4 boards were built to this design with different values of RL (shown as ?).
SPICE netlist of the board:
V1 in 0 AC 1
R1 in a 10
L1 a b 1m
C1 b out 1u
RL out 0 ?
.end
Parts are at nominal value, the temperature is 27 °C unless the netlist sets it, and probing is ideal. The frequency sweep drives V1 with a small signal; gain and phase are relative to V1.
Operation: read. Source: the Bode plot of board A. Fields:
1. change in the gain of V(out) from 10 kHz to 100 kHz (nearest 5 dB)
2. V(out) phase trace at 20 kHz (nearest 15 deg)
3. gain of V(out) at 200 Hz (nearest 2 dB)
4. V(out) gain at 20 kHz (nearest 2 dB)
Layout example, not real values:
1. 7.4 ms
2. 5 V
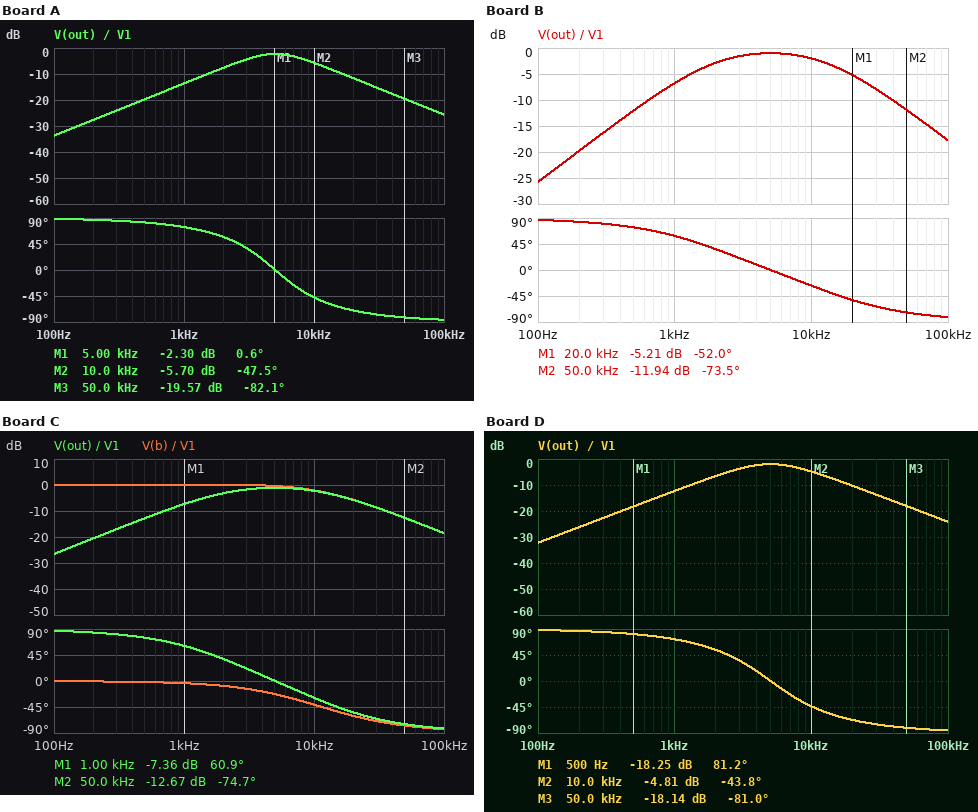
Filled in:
1. -20 dB
2. -75 deg
3. -28 dB
4. -12 dB
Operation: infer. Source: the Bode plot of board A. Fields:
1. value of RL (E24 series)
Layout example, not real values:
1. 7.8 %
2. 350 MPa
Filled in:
1. 33 Ω
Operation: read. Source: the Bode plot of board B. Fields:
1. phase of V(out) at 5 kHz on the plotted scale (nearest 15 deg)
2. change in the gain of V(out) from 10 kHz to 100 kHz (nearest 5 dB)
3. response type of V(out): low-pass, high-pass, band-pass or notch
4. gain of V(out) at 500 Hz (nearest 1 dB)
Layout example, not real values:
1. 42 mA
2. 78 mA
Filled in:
1. 0 deg
2. -15 dB
3. band-pass
4. -12 dB
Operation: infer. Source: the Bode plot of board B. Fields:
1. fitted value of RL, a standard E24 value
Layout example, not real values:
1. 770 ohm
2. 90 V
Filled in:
1. 82 Ω
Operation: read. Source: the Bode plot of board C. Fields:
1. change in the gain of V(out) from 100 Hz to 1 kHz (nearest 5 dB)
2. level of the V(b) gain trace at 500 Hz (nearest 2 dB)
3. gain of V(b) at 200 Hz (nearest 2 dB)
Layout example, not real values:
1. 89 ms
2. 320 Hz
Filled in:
1. 20 dB
2. 0 dB
3. 0 dB
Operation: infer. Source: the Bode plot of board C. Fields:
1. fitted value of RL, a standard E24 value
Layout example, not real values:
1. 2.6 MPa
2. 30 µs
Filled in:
1. 75 Ω
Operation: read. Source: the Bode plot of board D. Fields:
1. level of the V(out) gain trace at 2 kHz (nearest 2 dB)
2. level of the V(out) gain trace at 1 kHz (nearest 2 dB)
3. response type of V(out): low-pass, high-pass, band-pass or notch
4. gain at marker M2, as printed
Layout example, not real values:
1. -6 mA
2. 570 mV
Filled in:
1. -6 dB
2. -12 dB
3. band-pass
4. -4.81 dB
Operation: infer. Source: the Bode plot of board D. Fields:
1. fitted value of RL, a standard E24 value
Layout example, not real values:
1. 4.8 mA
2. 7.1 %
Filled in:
1. 39 Ω
